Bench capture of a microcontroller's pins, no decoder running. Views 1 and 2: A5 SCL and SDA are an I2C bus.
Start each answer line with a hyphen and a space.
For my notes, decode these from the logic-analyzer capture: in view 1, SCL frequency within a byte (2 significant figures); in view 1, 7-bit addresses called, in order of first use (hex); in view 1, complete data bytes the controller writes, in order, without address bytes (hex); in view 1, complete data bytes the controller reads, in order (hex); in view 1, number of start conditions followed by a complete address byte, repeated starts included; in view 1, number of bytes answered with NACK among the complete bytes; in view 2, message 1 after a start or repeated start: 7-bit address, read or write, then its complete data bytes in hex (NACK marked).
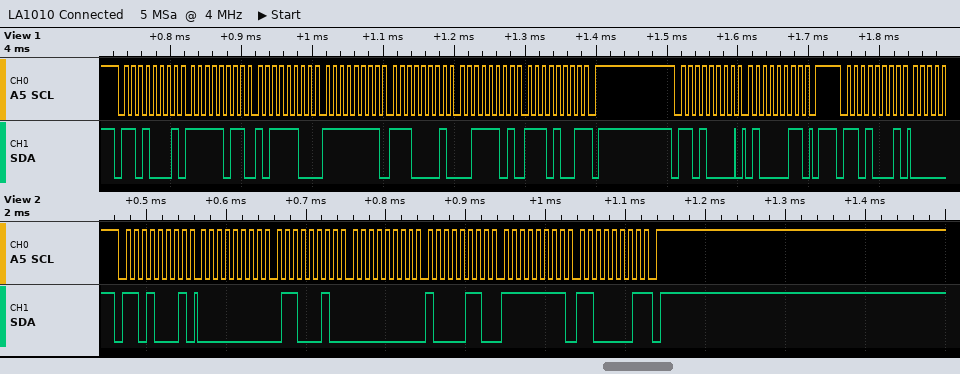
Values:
- 100 kHz
- 0x68
- 43
- FB BC FF E1 3D E9
- 3
- 1
- 0x68 read: 00 62 00 86 FF C1 NACK
